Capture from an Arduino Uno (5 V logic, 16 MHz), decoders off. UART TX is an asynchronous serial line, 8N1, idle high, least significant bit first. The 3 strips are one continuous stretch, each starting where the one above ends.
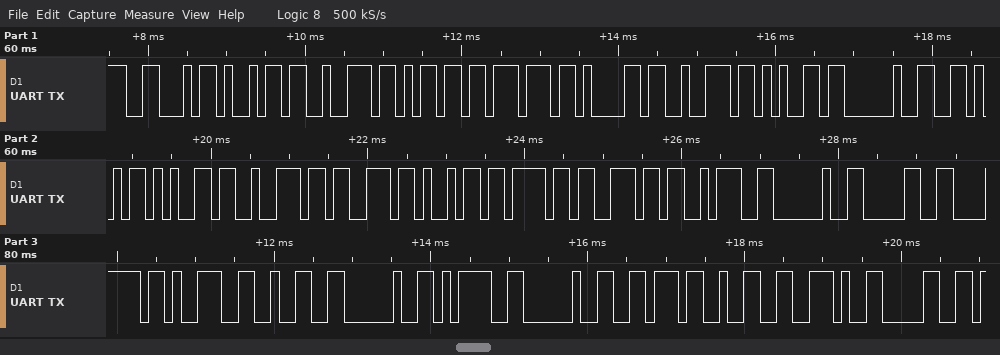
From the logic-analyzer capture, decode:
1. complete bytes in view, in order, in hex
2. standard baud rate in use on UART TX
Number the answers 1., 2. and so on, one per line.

1. 46 69 72 6D 77 61 72 65 20 56 65 72 73 69 6F 6E 3A 20 30 78 39 32 20 3D 20 76 32 2E 30
2. 9600 baud
